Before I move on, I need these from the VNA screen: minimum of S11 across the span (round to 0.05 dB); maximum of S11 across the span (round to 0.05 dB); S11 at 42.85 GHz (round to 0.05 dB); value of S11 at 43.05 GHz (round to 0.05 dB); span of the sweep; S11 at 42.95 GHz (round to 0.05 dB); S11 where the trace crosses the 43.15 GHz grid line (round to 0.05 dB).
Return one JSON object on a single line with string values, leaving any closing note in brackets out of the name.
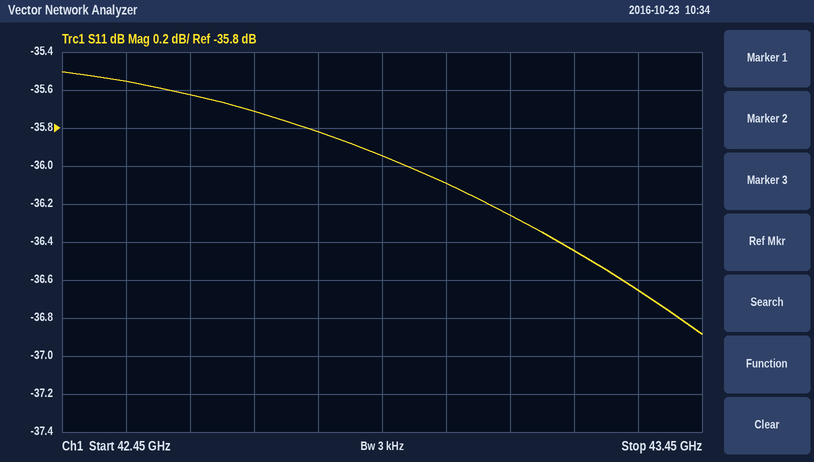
{"minimum of S11 across the span": "-36.90 dB", "maximum of S11 across the span": "-35.50 dB", "S11 at 42.85 GHz": "-35.80 dB", "value of S11 at 43.05 GHz": "-36.10 dB", "span of the sweep": "1 GHz", "S11 at 42.95 GHz": "-35.95 dB", "S11 where the trace crosses the 43.15 GHz grid line": "-36.25 dB"}
